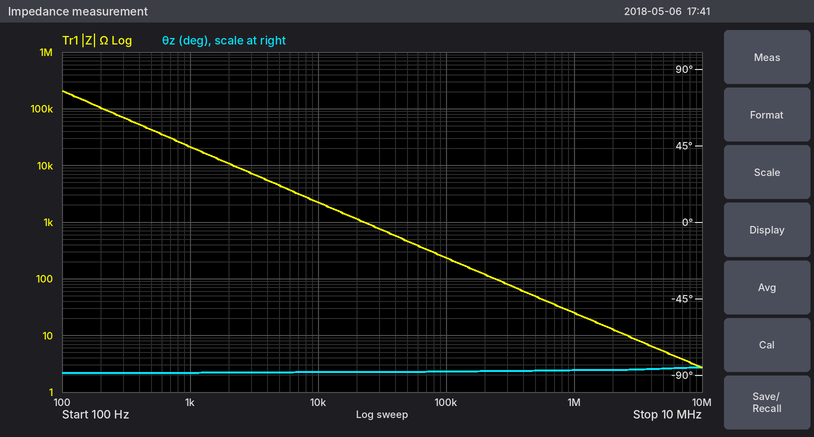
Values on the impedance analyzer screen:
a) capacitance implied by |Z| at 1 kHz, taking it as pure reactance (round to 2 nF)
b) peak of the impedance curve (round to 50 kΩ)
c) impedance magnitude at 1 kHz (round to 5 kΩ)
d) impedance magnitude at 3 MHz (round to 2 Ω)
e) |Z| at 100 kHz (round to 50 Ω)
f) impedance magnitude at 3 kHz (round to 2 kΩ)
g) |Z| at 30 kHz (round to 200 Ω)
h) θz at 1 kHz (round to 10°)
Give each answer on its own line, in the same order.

8 nF
200 kΩ
20 kΩ
8 Ω
250 Ω
8 kΩ
800 Ω
-90°
